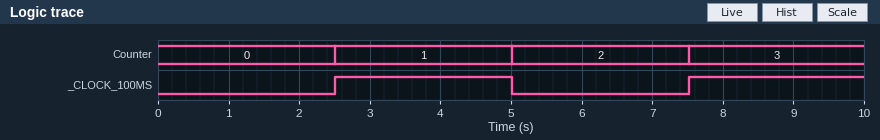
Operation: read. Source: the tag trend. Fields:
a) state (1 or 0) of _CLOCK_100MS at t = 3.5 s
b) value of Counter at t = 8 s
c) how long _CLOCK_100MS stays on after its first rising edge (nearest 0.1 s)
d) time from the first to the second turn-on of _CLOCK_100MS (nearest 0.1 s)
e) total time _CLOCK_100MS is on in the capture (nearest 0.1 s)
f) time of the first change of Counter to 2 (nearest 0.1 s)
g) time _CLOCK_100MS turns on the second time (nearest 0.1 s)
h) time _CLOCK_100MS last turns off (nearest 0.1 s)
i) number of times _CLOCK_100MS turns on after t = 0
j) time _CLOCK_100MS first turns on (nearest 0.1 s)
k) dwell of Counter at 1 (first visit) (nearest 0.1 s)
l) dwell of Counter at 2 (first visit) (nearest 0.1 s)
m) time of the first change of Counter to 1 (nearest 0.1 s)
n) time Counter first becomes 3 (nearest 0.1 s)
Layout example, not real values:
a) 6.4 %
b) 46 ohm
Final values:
a) 1
b) 3
c) 2.5 s
d) 5.0 s
e) 5.0 s
f) 5.0 s
g) 7.5 s
h) 5.0 s
i) 2
j) 2.5 s
k) 2.5 s
l) 2.5 s
m) 2.5 s
n) 7.5 s
